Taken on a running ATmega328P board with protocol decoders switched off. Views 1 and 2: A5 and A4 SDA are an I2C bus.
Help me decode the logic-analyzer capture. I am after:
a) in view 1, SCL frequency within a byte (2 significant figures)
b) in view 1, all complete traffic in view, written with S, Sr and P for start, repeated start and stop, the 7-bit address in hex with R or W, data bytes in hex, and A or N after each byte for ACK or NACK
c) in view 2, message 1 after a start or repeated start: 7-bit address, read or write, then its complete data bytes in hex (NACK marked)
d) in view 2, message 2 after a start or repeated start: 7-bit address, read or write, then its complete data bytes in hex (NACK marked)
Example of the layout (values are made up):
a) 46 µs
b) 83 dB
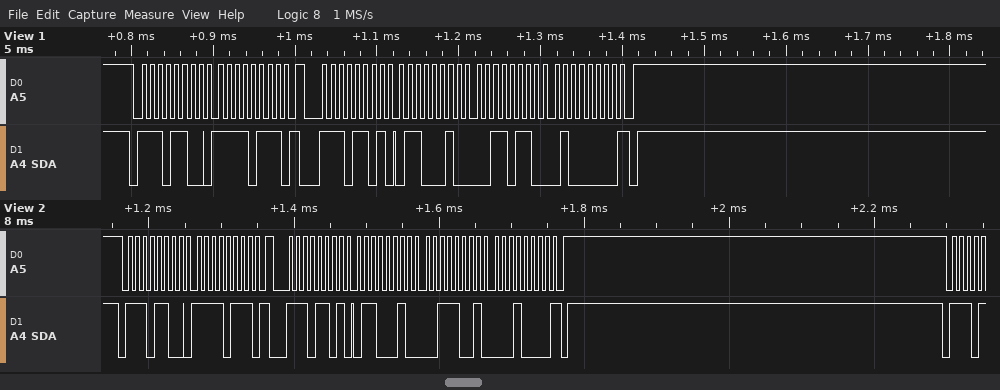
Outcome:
a) 100 kHz
b) S 76W A F7 A Sr 76R A 62 A 36 A 40 N P
c) 0x76 write: F7
d) 0x76 read: 62 39 10 NACK
